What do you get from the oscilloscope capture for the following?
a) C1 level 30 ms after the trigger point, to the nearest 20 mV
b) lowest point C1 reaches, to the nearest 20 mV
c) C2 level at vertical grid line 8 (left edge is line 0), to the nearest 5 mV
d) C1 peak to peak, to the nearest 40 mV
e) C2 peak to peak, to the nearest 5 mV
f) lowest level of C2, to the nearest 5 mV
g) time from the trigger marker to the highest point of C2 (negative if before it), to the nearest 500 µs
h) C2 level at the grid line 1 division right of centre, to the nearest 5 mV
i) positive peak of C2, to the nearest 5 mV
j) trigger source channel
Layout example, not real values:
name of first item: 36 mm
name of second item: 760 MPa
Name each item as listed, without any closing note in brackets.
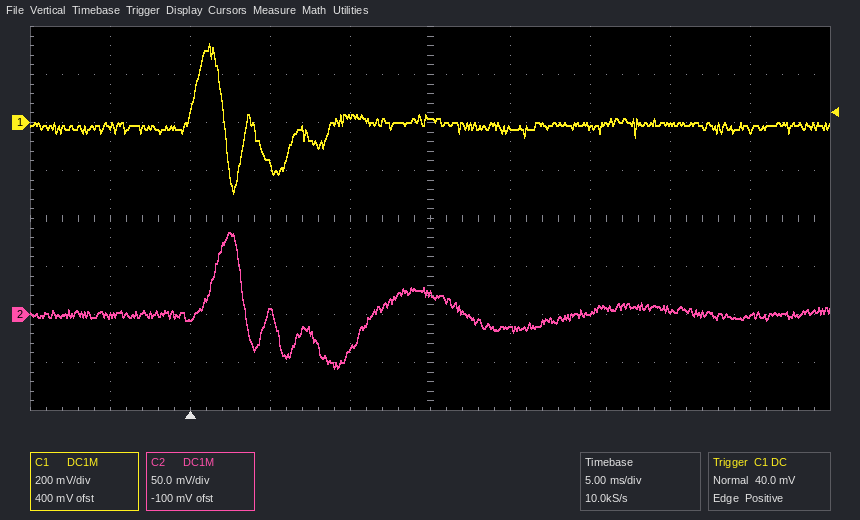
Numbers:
C1 level 30 ms after the trigger point, to the nearest 20 mV: 0 mV
lowest point C1 reaches, to the nearest 20 mV: -300 mV
C2 level at vertical grid line 8 (left edge is line 0), to the nearest 5 mV: 5 mV
C1 peak to peak, to the nearest 40 mV: 640 mV
C2 peak to peak, to the nearest 5 mV: 140 mV
lowest level of C2, to the nearest 5 mV: -55 mV
time from the trigger marker to the highest point of C2 (negative if before it), to the nearest 500 µs: +2.5 ms
C2 level at the grid line 1 division right of centre, to the nearest 5 mV: -15 mV
positive peak of C2, to the nearest 5 mV: 85 mV
trigger source channel: C1
